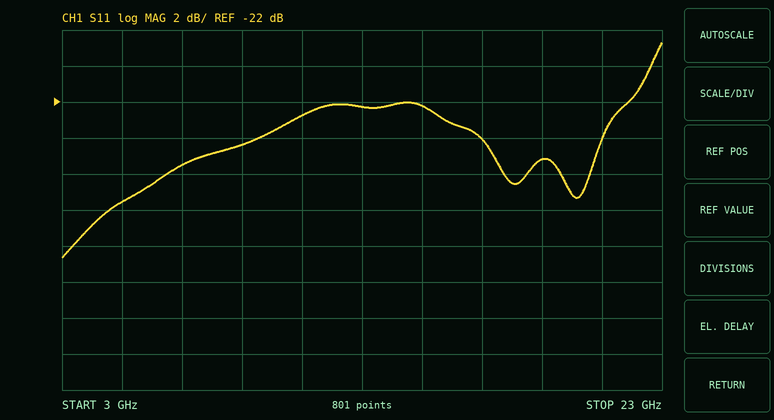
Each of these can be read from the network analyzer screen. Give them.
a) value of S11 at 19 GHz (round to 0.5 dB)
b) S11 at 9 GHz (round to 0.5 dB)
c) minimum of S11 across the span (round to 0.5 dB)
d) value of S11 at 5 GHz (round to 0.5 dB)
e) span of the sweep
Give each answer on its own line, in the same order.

-25.0 dB
-24.5 dB
-30.5 dB
-27.5 dB
20 GHz
